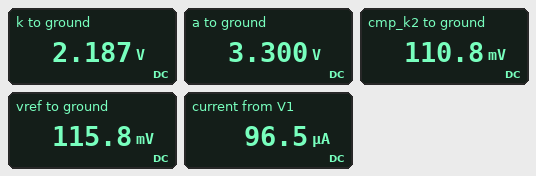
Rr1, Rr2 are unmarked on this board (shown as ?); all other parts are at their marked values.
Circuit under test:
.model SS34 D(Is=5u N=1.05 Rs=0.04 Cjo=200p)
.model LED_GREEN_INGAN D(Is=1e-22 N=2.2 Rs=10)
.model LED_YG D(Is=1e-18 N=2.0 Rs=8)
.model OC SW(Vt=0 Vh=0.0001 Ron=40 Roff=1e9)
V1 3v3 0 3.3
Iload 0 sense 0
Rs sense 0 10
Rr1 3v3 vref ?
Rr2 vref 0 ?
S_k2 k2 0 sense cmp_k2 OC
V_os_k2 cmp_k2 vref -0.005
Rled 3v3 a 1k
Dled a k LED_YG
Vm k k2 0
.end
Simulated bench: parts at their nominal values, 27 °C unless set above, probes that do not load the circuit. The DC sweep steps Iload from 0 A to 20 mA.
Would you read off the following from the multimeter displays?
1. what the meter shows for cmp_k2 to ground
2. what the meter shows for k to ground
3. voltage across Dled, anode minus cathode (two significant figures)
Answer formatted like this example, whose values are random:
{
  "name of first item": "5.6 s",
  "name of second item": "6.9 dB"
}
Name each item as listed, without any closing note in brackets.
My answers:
{
  "what the meter shows for cmp_k2 to ground": "110.8 mV",
  "what the meter shows for k to ground": "2.187 V",
  "voltage across Dled, anode minus cathode": "1.1 V"
}
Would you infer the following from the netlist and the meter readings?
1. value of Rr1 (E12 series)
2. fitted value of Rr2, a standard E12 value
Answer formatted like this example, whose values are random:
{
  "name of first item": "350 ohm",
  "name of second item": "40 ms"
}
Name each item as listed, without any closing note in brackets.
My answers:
{
  "value of Rr1": "33 kΩ",
  "fitted value of Rr2, a standard E12 value": "1.2 kΩ"
}
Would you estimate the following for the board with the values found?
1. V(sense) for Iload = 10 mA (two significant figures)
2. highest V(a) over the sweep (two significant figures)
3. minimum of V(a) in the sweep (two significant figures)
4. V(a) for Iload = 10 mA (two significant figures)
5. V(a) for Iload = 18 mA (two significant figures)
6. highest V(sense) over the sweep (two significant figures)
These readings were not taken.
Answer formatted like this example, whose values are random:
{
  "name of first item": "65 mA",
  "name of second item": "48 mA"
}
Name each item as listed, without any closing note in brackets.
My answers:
{
  "V(sense) for Iload = 10 mA": "100 mV",
  "highest V(a) over the sweep": "3.3 V",
  "minimum of V(a) in the sweep": "1.9 V",
  "V(a) for Iload = 10 mA": "3.3 V",
  "V(a) for Iload = 18 mA": "1.9 V",
  "highest V(sense) over the sweep": "200 mV"
}
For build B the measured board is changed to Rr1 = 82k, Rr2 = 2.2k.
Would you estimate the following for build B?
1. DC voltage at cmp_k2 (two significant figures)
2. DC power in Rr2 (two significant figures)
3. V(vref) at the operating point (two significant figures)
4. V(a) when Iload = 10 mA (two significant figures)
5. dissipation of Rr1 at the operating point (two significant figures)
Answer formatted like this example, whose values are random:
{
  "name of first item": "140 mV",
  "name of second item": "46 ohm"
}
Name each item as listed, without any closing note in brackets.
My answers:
{
  "DC voltage at cmp_k2": "81 mV",
  "DC power in Rr2": "3.4 µW",
  "V(vref) at the operating point": "86 mV",
  "V(a) when Iload = 10 mA": "1.9 V",
  "dissipation of Rr1 at the operating point": "130 µW"
}
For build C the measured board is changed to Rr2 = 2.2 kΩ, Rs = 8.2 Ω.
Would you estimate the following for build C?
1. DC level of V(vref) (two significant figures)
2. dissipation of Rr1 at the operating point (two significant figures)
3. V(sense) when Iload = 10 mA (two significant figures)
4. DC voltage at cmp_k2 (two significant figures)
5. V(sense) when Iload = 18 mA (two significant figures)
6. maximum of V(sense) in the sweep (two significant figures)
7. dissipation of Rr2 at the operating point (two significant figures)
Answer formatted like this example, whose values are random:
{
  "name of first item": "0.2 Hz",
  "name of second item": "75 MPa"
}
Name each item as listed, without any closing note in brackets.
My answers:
{
  "DC level of V(vref)": "210 mV",
  "dissipation of Rr1 at the operating point": "290 µW",
  "V(sense) when Iload = 10 mA": "82 mV",
  "DC voltage at cmp_k2": "200 mV",
  "V(sense) when Iload = 18 mA": "150 mV",
  "maximum of V(sense) in the sweep": "160 mV",
  "dissipation of Rr2 at the operating point": "19 µW"
}
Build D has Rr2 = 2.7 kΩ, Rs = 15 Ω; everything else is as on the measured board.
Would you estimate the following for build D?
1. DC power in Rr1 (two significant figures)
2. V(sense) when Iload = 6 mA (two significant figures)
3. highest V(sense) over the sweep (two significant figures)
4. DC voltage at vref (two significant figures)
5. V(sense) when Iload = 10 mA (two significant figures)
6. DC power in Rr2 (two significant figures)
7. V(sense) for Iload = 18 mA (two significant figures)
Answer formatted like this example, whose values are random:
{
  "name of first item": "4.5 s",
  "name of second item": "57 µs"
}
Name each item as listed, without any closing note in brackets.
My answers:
{
  "DC power in Rr1": "280 µW",
  "V(sense) when Iload = 6 mA": "90 mV",
  "highest V(sense) over the sweep": "300 mV",
  "DC voltage at vref": "250 mV",
  "V(sense) when Iload = 10 mA": "150 mV",
  "DC power in Rr2": "23 µW",
  "V(sense) for Iload = 18 mA": "270 mV"
}
